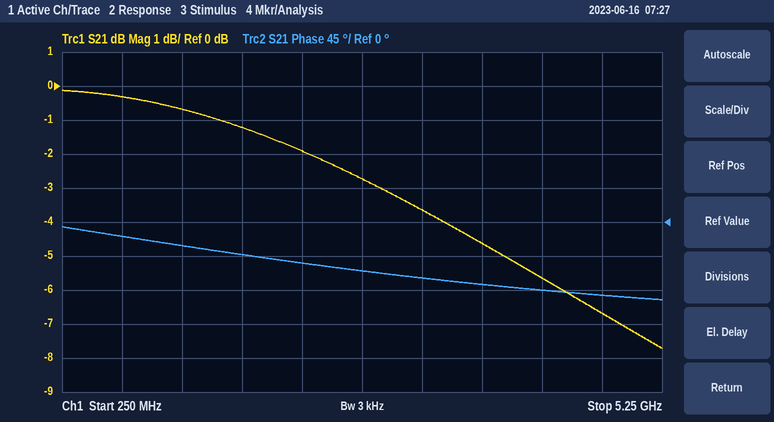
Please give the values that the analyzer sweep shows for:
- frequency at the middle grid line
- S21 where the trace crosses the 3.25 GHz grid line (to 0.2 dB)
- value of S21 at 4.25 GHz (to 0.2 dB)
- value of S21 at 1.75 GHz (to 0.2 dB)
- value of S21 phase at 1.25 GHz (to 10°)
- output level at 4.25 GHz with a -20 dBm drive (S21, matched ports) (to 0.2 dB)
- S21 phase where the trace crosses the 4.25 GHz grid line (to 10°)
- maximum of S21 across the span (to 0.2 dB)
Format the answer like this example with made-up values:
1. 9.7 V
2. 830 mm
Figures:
1. 2.75 GHz
2. -3.6 dB
3. -5.6 dB
4. -1.2 dB
5. -30°
6. -25.6 dBm
7. -90°
8. -0.2 dB
